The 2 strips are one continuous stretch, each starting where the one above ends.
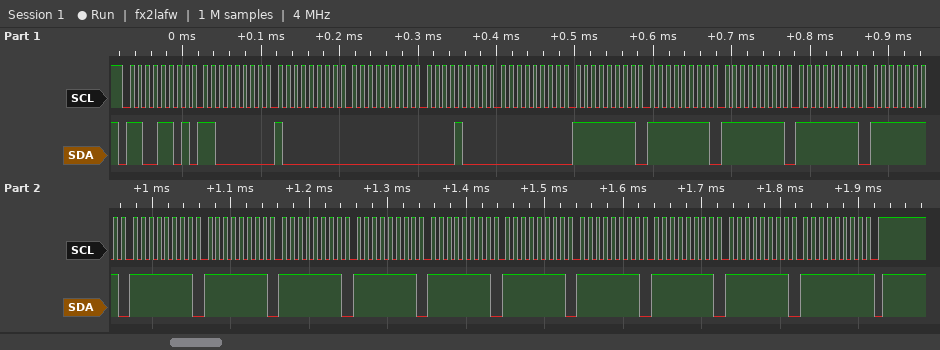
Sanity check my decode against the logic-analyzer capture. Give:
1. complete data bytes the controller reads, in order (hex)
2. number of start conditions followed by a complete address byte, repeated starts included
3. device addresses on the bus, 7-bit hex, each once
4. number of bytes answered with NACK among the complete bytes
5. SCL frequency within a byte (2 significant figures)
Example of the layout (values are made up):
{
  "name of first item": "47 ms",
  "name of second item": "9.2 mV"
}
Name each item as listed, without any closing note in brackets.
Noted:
{
  "complete data bytes the controller reads, in order": "C0 80 00 08 00 FF FF FF FF FF FF FF FF FF FF FF FF FF FF FF",
  "number of start conditions followed by a complete address byte, repeated starts included": "1",
  "device addresses on the bus, 7-bit hex, each once": "0x66",
  "number of bytes answered with NACK among the complete bytes": "1",
  "SCL frequency within a byte": "100 kHz"
}
